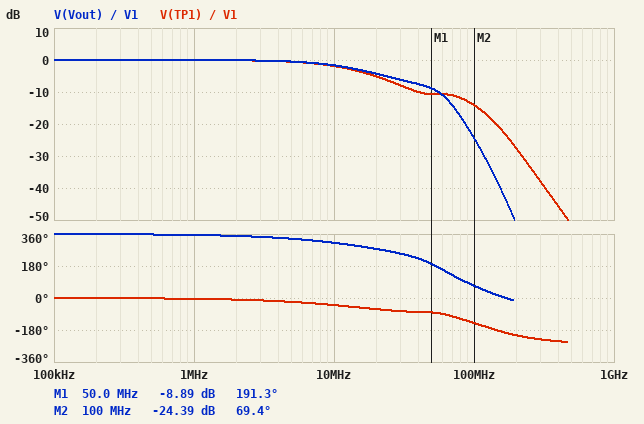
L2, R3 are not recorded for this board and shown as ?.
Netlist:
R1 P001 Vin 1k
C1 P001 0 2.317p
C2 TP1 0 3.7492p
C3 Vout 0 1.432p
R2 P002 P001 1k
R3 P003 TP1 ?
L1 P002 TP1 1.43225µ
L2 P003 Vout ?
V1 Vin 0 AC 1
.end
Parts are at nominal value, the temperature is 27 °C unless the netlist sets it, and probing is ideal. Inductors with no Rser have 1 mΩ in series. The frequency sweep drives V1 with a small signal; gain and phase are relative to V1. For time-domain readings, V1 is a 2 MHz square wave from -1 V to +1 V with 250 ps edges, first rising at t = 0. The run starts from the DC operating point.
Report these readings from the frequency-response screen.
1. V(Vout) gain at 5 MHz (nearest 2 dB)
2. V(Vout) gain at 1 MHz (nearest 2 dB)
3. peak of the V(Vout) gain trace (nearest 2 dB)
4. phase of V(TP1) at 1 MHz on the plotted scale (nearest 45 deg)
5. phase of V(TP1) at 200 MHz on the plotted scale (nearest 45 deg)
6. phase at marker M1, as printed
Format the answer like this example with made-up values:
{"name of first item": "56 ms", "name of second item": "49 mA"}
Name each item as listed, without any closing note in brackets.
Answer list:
{"V(Vout) gain at 5 MHz": "0 dB", "V(Vout) gain at 1 MHz": "0 dB", "peak of the V(Vout) gain trace": "0 dB", "phase of V(TP1) at 1 MHz on the plotted scale": "0 deg", "phase of V(TP1) at 200 MHz on the plotted scale": "-225 deg", "phase at marker M1, as printed": "191.3 deg"}
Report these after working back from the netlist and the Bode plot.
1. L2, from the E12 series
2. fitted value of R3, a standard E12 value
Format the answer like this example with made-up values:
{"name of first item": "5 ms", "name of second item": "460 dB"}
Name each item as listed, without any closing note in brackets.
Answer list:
{"L2, from the E12 series": "6.8 µH", "fitted value of R3, a standard E12 value": "1.8 kΩ"}
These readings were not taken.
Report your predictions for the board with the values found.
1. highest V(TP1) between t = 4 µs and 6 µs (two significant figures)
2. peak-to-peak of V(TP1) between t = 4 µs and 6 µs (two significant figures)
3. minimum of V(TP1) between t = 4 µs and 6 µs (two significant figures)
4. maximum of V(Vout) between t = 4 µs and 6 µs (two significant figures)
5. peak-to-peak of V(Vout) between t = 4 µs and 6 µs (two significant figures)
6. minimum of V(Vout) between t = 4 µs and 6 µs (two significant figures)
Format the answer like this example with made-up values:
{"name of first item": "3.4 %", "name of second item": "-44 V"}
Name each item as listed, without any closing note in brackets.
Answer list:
{"highest V(TP1) between t = 4 µs and 6 µs": "1.0 V", "peak-to-peak of V(TP1) between t = 4 µs and 6 µs": "2.0 V", "minimum of V(TP1) between t = 4 µs and 6 µs": "-1.0 V", "maximum of V(Vout) between t = 4 µs and 6 µs": "1.0 V", "peak-to-peak of V(Vout) between t = 4 µs and 6 µs": "2.0 V", "minimum of V(Vout) between t = 4 µs and 6 µs": "-1.0 V"}
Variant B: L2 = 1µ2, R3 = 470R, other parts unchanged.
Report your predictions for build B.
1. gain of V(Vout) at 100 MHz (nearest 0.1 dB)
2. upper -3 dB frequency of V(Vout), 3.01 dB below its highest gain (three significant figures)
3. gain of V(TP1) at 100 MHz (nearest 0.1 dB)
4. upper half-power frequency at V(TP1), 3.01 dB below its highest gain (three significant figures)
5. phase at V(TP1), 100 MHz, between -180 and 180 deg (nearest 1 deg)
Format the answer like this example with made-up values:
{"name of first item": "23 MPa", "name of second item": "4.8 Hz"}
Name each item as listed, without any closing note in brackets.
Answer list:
{"gain of V(Vout) at 100 MHz": "-13.8 dB", "upper -3 dB frequency of V(Vout), 3.01 dB below its highest gain": "14.5 MHz", "gain of V(TP1) at 100 MHz": "-19.3 dB", "upper half-power frequency at V(TP1), 3.01 dB below its highest gain": "14.2 MHz", "phase at V(TP1), 100 MHz, between -180 and 180 deg": "-131 deg"}
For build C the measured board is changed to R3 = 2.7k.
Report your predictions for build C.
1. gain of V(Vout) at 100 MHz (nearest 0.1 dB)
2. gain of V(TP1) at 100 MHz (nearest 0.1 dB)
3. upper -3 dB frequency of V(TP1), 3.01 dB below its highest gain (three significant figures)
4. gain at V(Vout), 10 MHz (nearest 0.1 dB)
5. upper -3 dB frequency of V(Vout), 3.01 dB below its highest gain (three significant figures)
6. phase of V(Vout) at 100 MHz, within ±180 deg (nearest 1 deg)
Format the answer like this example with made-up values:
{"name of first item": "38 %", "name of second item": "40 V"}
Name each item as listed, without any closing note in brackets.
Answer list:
{"gain of V(Vout) at 100 MHz": "-25.8 dB", "gain of V(TP1) at 100 MHz": "-14.3 dB", "upper -3 dB frequency of V(TP1), 3.01 dB below its highest gain": "13.3 MHz", "gain at V(Vout), 10 MHz": "-1.9 dB", "upper -3 dB frequency of V(Vout), 3.01 dB below its highest gain": "13.7 MHz", "phase of V(Vout) at 100 MHz, within ±180 deg": "80 deg"}
